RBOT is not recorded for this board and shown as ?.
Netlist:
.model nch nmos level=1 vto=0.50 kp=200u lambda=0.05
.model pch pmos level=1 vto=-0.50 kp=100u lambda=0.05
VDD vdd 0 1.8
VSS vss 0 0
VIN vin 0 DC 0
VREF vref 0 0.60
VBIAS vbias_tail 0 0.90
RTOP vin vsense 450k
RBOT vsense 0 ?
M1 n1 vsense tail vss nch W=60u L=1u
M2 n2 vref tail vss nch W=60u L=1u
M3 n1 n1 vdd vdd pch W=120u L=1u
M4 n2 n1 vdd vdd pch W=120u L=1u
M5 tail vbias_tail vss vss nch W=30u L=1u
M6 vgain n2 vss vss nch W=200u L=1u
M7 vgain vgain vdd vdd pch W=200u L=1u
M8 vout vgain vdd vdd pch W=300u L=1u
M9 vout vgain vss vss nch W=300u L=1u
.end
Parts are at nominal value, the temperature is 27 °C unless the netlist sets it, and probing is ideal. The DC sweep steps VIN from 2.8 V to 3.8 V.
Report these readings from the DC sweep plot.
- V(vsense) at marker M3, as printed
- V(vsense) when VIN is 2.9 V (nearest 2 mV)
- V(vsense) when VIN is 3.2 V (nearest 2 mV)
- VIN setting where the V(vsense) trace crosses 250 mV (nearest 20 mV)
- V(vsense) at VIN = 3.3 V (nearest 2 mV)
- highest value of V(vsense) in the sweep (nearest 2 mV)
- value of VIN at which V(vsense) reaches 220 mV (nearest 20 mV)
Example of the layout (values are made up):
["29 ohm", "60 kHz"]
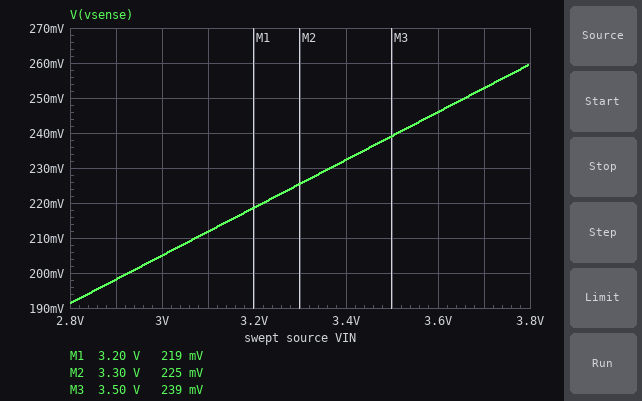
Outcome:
["239 mV", "198 mV", "218 mV", "3.66 V", "226 mV", "260 mV", "3.22 V"]
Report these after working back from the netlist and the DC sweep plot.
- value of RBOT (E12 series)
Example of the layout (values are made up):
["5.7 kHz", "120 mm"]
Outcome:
["33 kΩ"]
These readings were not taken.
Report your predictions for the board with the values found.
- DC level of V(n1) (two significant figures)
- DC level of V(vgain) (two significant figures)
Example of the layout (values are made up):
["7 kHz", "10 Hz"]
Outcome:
["1.3 V", "1.3 V"]
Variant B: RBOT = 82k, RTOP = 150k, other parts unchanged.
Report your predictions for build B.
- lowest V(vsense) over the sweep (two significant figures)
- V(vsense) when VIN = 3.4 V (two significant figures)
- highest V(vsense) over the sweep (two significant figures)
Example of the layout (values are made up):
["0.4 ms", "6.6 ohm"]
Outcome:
["990 mV", "1.2 V", "1.3 V"]
